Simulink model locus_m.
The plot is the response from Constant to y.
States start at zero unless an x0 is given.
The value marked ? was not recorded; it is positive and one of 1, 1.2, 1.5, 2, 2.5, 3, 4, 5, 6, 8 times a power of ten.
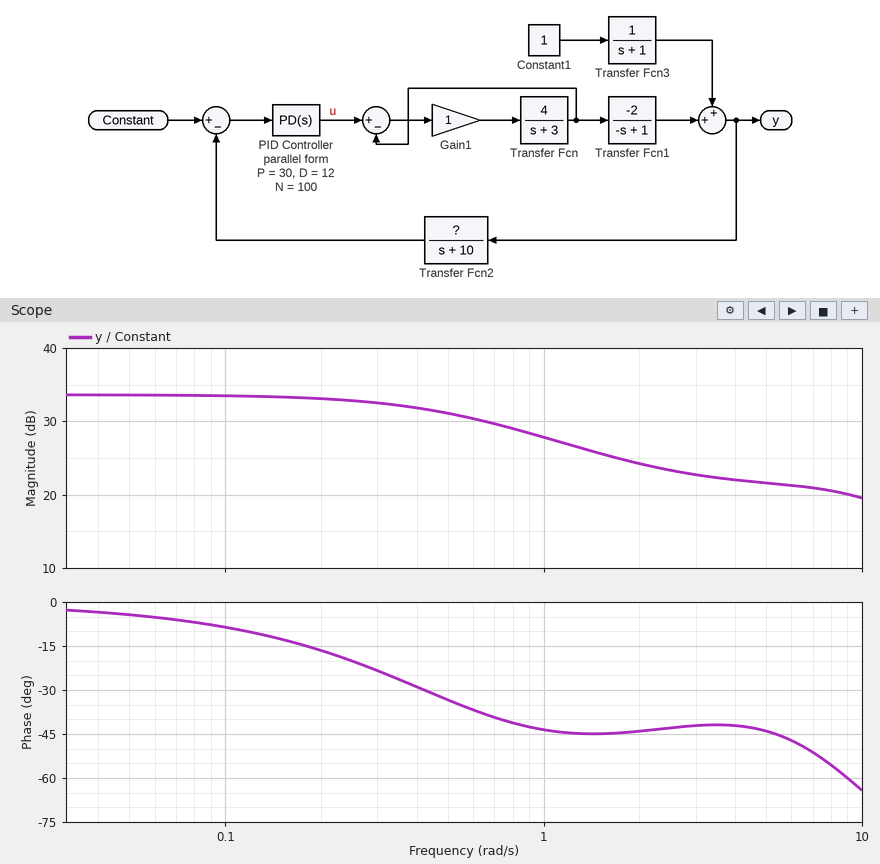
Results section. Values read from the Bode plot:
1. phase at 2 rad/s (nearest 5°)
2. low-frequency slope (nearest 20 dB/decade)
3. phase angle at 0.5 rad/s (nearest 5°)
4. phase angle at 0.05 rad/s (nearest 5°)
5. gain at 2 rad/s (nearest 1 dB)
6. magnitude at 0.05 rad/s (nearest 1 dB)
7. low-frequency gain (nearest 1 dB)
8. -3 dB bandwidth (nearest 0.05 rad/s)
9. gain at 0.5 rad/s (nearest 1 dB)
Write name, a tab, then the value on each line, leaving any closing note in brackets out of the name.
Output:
phase at 2 rad/s	-45°
low-frequency slope	0 dB/decade
phase angle at 0.5 rad/s	-35°
phase angle at 0.05 rad/s	-5°
gain at 2 rad/s	24 dB
magnitude at 0.05 rad/s	34 dB
low-frequency gain	34 dB
-3 dB bandwidth	0.55 rad/s
gain at 0.5 rad/s	31 dB
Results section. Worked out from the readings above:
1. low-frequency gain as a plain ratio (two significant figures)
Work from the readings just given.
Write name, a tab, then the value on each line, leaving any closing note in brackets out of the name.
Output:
low-frequency gain as a plain ratio	50
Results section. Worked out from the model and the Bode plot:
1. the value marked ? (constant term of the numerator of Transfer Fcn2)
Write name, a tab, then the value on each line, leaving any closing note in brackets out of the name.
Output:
the value marked ?	0.5
